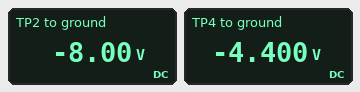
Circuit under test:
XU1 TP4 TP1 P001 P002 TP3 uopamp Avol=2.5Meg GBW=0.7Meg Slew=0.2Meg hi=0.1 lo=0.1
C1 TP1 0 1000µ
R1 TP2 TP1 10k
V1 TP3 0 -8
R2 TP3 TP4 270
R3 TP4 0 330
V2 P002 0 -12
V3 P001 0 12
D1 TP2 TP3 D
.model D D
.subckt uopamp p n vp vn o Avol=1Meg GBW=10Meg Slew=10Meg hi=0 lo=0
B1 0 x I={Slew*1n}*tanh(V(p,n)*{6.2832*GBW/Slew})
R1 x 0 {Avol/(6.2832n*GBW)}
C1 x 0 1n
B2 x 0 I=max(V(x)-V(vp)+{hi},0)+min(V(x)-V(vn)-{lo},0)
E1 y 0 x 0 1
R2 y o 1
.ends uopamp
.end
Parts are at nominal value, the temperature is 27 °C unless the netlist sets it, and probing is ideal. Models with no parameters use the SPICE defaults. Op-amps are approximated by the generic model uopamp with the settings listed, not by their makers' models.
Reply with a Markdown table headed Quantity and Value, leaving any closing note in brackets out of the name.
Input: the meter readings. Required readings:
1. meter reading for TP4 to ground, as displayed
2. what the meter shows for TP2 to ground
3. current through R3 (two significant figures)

| Quantity | Value |
|---|---|
| meter reading for TP4 to ground, as displayed | -4.400 V |
| what the meter shows for TP2 to ground | -8.00 V |
| current through R3 | 13 mA |
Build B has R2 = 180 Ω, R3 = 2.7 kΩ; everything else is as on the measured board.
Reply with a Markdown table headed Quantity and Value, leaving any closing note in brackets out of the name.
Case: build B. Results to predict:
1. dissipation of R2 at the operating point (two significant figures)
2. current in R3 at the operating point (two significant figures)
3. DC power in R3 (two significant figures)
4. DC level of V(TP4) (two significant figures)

| Quantity | Value |
|---|---|
| dissipation of R2 at the operating point | 1.4 mW |
| current in R3 at the operating point | 2.8 mA |
| DC power in R3 | 21 mW |
| DC level of V(TP4) | -7.5 V |
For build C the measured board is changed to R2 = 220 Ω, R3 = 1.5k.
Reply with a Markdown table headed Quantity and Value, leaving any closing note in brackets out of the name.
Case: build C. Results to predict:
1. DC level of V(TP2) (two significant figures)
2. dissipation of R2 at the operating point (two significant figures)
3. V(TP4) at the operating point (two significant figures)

| Quantity | Value |
|---|---|
| DC level of V(TP2) | -8.0 V |
| dissipation of R2 at the operating point | 4.8 mW |
| V(TP4) at the operating point | -7.0 V |
